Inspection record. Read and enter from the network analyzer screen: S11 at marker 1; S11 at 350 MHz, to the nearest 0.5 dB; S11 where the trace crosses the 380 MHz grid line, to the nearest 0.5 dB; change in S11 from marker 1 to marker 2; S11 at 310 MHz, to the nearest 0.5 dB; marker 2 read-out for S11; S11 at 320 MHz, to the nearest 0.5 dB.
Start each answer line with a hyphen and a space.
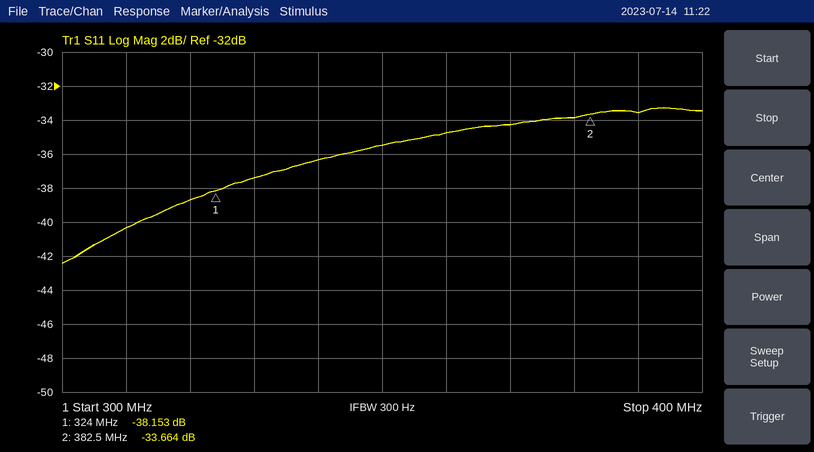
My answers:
- -38.153 dB
- -35.5 dB
- -34.0 dB
- 4.489 dB
- -40.5 dB
- -33.664 dB
- -38.5 dB
